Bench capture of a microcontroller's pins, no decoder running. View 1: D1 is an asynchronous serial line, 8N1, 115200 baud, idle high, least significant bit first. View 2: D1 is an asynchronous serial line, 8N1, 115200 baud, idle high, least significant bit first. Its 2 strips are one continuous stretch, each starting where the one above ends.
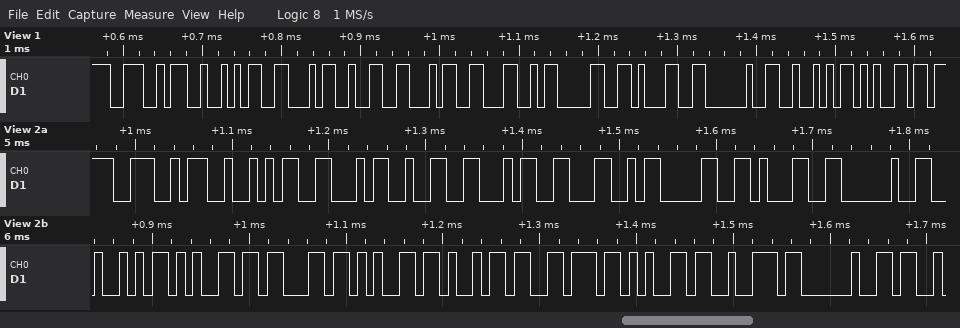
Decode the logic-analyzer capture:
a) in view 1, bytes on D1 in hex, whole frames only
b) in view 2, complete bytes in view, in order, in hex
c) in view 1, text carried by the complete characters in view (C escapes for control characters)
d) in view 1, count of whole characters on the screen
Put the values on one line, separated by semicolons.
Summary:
4E 52 46 32 34 4C 30 31 20 52 65; 4E 52 46 32 34 4C 30 31 20 52 65 63 65 69 76 65 72 20; "NRF24L01 Re"; 11
